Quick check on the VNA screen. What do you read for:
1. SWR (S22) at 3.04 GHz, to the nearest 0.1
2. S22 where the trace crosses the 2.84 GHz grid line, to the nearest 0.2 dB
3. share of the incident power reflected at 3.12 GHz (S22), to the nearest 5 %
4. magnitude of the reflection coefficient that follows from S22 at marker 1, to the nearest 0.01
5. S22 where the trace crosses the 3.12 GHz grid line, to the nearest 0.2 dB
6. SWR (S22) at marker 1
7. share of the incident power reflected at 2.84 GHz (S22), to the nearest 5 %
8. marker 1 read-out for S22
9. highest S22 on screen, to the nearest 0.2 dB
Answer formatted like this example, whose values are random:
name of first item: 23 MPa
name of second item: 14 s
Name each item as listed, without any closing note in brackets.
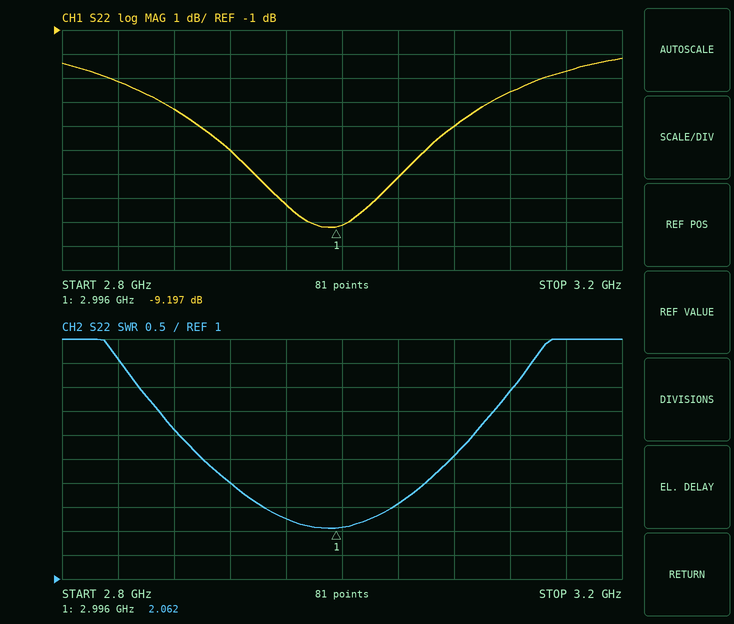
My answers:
SWR (S22) at 3.04 GHz, to the nearest 0.1: 2.6
S22 where the trace crosses the 2.84 GHz grid line, to the nearest 0.2 dB: -3.2 dB
share of the incident power reflected at 3.12 GHz (S22), to the nearest 5 %: 45 %
magnitude of the reflection coefficient that follows from S22 at marker 1, to the nearest 0.01: 0.35
S22 where the trace crosses the 3.12 GHz grid line, to the nearest 0.2 dB: -3.6 dB
SWR (S22) at marker 1: 2.062
share of the incident power reflected at 2.84 GHz (S22), to the nearest 5 %: 50 %
marker 1 read-out for S22: -9.197 dB
highest S22 on screen, to the nearest 0.2 dB: -2.2 dB
